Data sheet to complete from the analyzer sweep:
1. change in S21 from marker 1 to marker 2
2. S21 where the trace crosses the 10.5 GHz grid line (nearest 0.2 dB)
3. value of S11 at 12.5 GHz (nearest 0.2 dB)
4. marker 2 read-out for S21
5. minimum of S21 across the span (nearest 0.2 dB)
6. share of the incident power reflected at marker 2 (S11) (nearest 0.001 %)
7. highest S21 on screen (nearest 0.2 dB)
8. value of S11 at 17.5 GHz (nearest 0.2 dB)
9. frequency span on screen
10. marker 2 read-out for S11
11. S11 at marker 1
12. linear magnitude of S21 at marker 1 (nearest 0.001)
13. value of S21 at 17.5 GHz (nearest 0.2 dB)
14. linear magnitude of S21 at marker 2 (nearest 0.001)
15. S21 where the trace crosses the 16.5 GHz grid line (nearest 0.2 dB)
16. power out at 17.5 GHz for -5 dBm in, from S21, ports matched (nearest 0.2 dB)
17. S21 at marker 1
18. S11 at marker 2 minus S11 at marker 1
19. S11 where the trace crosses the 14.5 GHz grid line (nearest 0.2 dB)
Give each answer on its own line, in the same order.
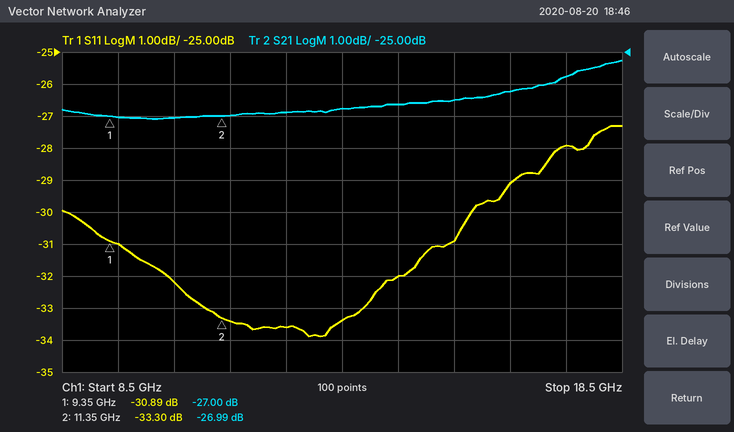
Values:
0.01 dB
-27.0 dB
-33.6 dB
-26.99 dB
-27.0 dB
0.047 %
-25.2 dB
-28.0 dB
10 GHz
-33.30 dB
-30.89 dB
0.045
-25.8 dB
0.045
-26.2 dB
-30.8 dBm
-27.00 dB
-2.41 dB
-32.0 dB
